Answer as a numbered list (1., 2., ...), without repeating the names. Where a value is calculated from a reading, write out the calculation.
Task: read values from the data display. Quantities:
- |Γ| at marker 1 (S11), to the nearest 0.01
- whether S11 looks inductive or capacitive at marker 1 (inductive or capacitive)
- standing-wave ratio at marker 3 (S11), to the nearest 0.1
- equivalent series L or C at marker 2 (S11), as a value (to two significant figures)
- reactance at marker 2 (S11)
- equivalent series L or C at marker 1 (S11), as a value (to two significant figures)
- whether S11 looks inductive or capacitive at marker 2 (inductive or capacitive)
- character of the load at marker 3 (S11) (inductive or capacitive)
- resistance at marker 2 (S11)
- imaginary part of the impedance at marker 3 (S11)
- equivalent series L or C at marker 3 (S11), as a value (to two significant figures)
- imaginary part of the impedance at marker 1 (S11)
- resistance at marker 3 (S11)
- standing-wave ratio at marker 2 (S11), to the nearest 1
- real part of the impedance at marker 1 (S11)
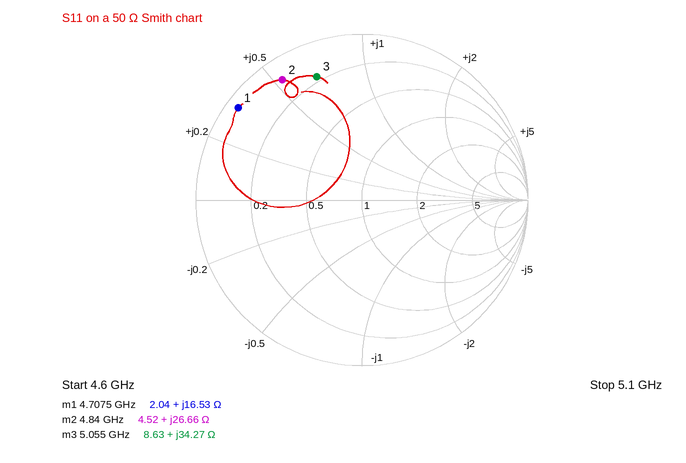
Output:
1. 0.93
2. inductive
3. 8.6
4. L = 26.66 Ω/(2π × 4.84 GHz) ≈ 877 pH, so 880 pH to two significant figures
5. +26.66 Ω
6. L = 16.53 Ω/(2π × 4.7075 GHz) ≈ 559 pH, so 560 pH to two significant figures
7. inductive
8. inductive
9. 4.52 Ω
10. +34.27 Ω
11. L = 34.27 Ω/(2π × 5.055 GHz) ≈ 1.1 nH
12. +16.53 Ω
13. 8.63 Ω
14. 14
15. 2.04 Ω
